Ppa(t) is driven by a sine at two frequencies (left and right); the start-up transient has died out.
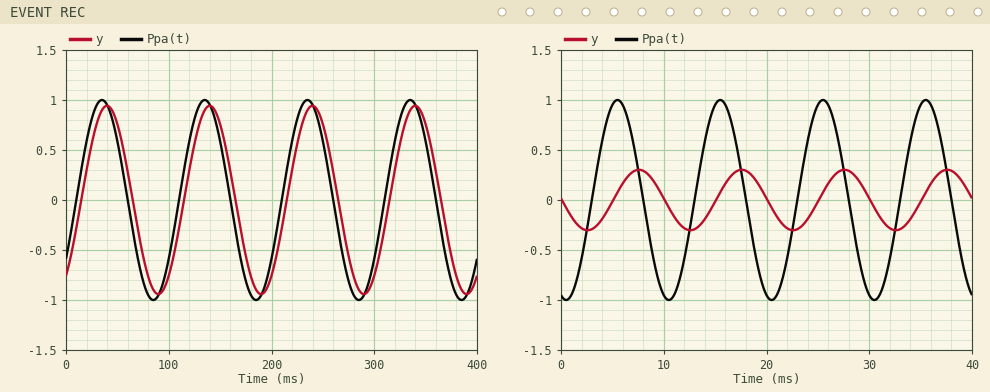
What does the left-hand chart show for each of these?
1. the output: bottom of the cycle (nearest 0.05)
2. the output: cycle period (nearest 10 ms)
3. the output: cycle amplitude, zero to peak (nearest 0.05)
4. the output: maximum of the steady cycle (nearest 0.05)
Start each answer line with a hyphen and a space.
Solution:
- -0.95
- 100 ms
- 0.95
- 0.95
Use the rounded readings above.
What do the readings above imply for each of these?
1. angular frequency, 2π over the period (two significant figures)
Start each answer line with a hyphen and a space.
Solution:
- 0.063 rad/ms
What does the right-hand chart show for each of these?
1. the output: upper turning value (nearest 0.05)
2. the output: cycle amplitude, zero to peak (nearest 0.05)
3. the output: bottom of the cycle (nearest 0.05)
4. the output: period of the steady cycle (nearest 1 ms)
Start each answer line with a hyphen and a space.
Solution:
- 0.30
- 0.30
- -0.30
- 10 ms
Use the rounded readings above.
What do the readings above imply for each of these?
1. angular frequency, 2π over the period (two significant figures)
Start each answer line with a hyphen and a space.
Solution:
- 0.63 rad/ms
